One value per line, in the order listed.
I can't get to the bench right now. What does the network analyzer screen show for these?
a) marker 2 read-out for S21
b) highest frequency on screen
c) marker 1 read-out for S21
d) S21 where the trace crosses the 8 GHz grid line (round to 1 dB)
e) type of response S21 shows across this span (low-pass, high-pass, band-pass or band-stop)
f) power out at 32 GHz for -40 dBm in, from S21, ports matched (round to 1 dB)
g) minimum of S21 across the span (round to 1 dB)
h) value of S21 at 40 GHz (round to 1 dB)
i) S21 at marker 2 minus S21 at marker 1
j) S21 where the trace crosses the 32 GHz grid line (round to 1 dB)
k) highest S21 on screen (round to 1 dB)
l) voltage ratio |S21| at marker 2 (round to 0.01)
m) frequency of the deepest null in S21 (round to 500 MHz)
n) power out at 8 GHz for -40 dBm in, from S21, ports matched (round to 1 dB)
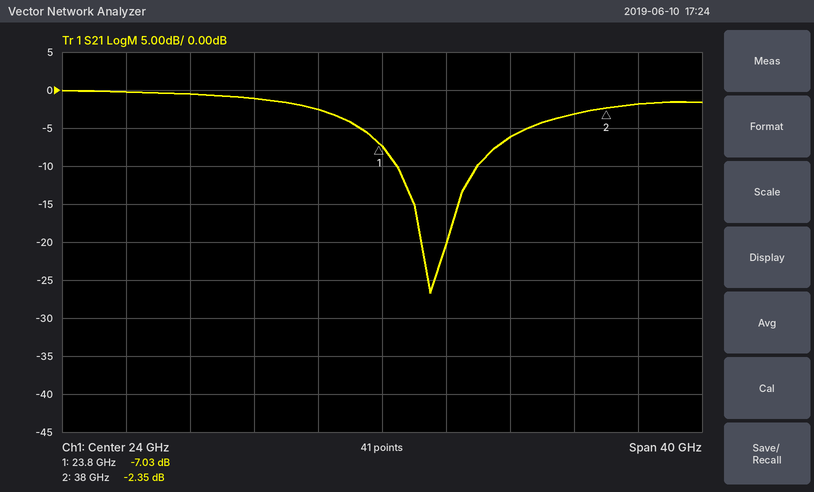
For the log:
-2.35 dB
44 GHz
-7.03 dB
0 dB
band-stop
-46 dBm
-27 dB
-2 dB
4.68 dB
-6 dB
0 dB
0.76
27.0 GHz
-40 dBm
